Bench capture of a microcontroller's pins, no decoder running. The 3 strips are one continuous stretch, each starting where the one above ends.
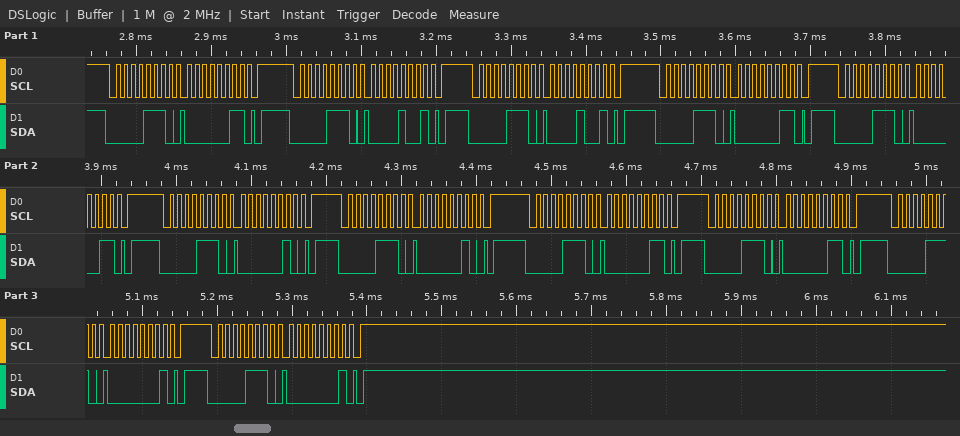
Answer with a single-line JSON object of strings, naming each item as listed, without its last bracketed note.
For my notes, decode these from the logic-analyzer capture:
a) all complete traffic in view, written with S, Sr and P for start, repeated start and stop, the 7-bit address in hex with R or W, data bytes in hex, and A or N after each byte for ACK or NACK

{"all complete traffic in view, written with S, Sr and P for start, repeated start and stop, the 7-bit address in hex with R or W, data bytes in hex, and A or N after each byte for ACK or NACK": "S 07W A 03 A P S 07W A 09 A P S 07W A 09 A P S 07W A 03 A P S 07W A 03 A P S 07W A 02 A P S 07W A 02 A P S 07W A 03 A P S 07W A 03 A P S 07W A 01 A P S 07W A 01 A P"}
